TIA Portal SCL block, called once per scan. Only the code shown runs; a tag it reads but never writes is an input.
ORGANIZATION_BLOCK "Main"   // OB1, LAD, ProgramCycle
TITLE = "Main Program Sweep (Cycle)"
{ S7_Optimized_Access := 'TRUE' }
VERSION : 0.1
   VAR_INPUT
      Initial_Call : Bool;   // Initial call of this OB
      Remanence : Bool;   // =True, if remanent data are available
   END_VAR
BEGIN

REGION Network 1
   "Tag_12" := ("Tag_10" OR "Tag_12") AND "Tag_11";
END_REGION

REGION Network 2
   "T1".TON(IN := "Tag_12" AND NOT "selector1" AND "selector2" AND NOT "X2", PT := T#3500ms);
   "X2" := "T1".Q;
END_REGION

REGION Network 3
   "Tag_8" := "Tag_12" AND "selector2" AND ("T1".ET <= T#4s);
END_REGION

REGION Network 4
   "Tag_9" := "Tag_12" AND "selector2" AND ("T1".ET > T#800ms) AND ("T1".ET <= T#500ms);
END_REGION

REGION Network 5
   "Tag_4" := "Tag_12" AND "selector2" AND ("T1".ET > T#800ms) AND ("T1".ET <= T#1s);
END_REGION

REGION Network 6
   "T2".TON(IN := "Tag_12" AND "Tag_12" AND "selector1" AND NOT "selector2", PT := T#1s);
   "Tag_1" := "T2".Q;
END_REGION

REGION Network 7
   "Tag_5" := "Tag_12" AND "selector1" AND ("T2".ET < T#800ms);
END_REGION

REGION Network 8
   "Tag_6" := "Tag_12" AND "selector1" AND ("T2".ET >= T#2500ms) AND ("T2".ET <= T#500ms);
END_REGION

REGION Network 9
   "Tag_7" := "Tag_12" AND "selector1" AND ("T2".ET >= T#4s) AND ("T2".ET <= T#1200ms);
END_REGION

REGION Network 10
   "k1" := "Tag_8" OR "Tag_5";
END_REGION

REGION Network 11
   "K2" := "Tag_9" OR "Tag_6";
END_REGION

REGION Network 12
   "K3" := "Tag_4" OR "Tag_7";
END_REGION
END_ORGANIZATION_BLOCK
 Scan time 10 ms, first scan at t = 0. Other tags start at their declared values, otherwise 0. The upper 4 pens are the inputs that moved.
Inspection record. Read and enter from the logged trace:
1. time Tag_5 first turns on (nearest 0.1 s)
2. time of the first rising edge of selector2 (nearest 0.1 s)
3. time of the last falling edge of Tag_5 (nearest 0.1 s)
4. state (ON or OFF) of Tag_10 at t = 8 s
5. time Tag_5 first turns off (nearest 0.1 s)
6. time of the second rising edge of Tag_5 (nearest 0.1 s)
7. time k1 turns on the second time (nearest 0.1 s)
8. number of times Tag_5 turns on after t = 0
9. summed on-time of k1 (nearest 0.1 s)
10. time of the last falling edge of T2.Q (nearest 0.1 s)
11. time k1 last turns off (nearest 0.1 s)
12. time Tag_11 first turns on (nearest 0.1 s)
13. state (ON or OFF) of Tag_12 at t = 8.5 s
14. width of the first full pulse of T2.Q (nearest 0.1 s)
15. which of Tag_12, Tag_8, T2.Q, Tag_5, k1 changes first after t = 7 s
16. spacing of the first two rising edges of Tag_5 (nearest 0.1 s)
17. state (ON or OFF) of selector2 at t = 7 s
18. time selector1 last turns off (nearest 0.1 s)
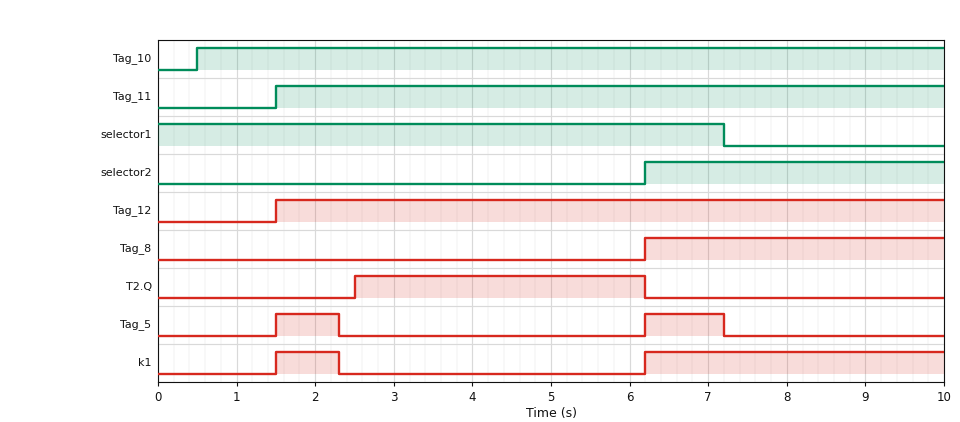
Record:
1.5 s
6.2 s
7.2 s
ON
2.3 s
6.2 s
6.2 s
2
4.6 s
6.2 s
2.3 s
1.5 s
ON
3.7 s
Tag_5
4.7 s
ON
7.2 s
